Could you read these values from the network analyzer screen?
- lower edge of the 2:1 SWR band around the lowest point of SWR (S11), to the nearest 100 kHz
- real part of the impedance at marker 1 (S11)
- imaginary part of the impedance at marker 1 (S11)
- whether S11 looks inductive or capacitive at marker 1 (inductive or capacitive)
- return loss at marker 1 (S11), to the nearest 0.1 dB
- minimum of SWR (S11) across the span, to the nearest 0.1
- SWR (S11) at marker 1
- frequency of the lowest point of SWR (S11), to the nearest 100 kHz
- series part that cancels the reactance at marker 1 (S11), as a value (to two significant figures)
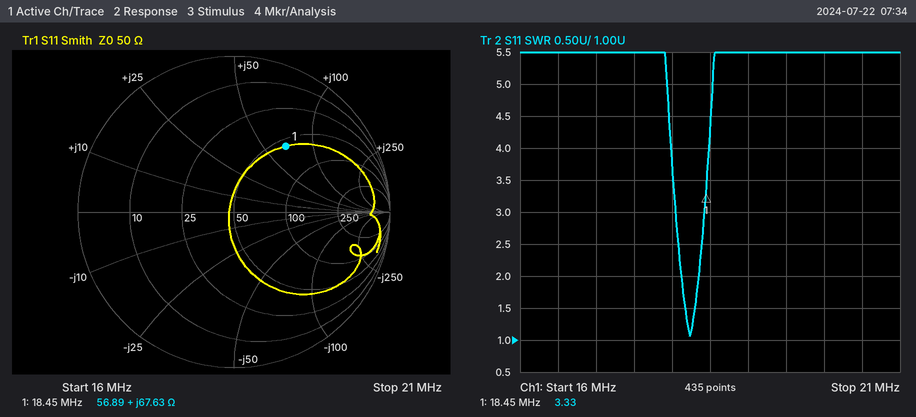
18.1 MHz
56.89 Ω
+67.63 Ω
inductive
5.4 dB
1.1
3.33
18.2 MHz
130 pF
